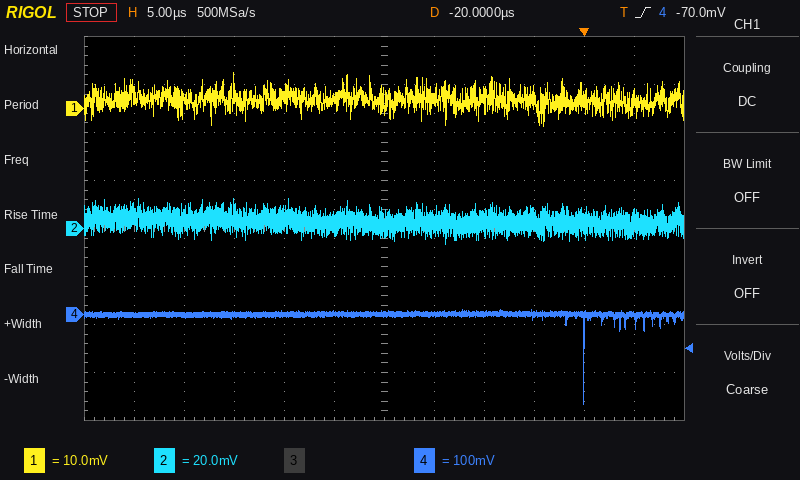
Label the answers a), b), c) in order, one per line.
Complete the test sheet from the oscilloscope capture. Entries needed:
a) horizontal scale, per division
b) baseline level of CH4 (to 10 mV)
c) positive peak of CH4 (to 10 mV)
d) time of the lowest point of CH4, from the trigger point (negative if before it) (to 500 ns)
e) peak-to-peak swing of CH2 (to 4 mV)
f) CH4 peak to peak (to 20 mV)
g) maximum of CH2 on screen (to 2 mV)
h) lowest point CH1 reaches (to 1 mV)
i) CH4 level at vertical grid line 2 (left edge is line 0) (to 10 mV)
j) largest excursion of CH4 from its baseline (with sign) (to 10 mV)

a) 5 µs
b) 0 mV
c) 10 mV
d) 0.0 µs
e) 20 mV
f) 200 mV
g) 12 mV
h) -4 mV
i) 0 mV
j) -190 mV
